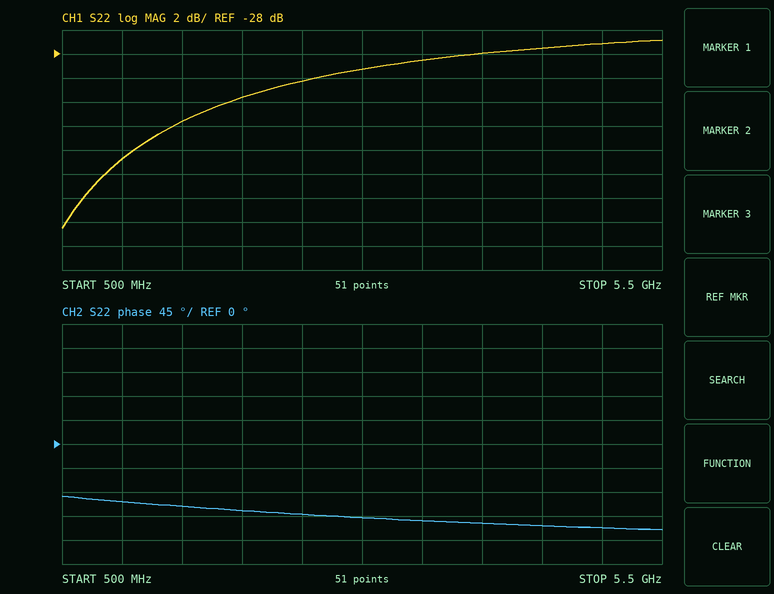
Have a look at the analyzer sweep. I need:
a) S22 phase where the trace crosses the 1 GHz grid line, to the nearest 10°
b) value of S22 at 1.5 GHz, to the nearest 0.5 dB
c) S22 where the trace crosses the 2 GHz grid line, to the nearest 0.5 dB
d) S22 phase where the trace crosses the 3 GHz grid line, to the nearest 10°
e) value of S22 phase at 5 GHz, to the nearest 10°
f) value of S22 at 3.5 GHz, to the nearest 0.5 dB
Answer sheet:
-110°
-33.5 dB
-31.5 dB
-140°
-160°
-28.5 dB
